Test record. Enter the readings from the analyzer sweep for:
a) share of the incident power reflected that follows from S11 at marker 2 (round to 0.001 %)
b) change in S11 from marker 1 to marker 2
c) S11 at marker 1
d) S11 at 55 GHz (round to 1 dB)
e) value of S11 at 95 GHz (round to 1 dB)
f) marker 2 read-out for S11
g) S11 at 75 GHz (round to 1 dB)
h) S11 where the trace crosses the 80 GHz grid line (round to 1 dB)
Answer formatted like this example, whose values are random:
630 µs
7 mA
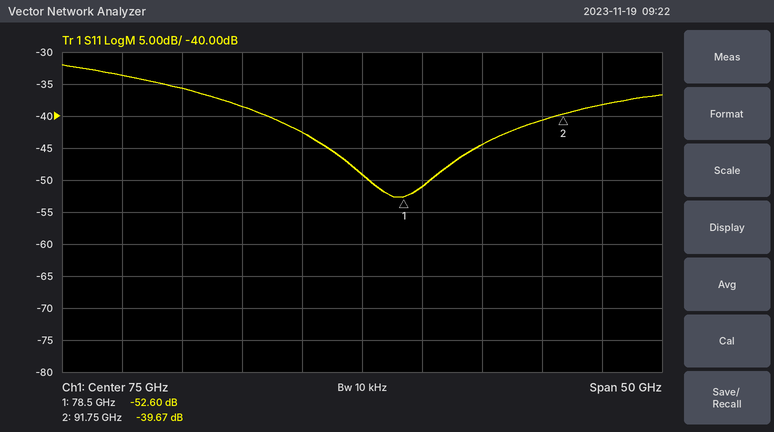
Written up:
0.011 %
12.93 dB
-52.60 dB
-34 dB
-38 dB
-39.67 dB
-49 dB
-51 dB
